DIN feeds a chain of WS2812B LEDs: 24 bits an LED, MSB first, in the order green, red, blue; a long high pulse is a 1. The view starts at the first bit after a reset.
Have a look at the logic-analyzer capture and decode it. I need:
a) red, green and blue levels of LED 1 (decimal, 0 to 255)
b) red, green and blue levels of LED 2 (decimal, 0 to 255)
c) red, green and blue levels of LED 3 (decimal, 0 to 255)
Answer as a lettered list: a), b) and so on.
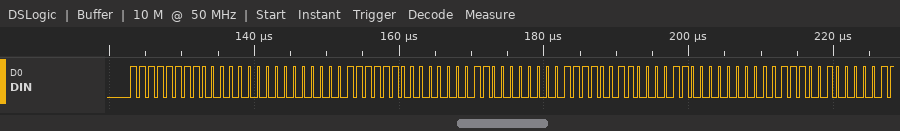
a) 0, 255, 0
b) 3, 252, 0
c) 12, 243, 0
